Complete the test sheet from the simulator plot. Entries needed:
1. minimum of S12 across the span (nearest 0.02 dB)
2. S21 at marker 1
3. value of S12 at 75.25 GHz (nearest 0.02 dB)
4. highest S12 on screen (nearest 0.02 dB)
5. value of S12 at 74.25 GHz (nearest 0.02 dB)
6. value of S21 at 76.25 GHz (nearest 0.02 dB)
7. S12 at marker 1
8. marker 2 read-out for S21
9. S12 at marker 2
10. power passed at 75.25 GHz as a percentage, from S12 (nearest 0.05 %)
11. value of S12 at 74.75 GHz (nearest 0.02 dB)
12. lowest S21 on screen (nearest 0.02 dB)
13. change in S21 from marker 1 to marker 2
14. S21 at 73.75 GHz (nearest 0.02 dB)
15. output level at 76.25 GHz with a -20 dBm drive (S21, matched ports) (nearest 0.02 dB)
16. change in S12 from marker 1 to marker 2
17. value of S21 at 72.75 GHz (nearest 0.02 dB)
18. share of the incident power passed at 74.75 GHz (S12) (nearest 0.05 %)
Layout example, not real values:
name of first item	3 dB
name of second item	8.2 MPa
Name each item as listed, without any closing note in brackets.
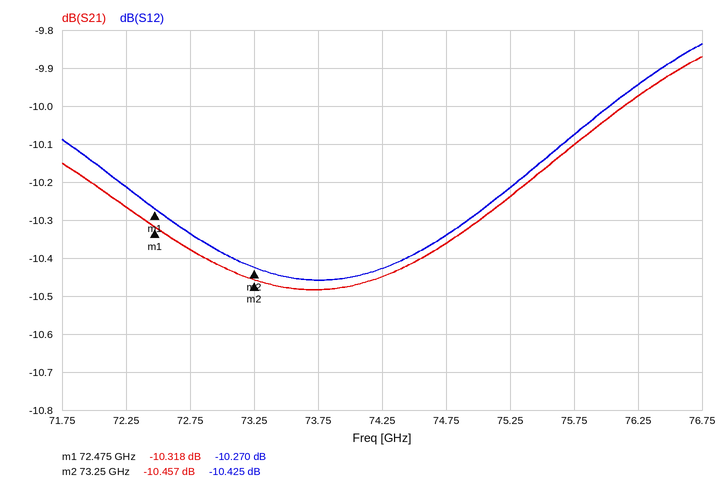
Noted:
minimum of S12 across the span	-10.46 dB
S21 at marker 1	-10.318 dB
value of S12 at 75.25 GHz	-10.22 dB
highest S12 on screen	-9.84 dB
value of S12 at 74.25 GHz	-10.42 dB
value of S21 at 76.25 GHz	-9.98 dB
S12 at marker 1	-10.270 dB
marker 2 read-out for S21	-10.457 dB
S12 at marker 2	-10.425 dB
power passed at 75.25 GHz as a percentage, from S12	9.50 %
value of S12 at 74.75 GHz	-10.34 dB
lowest S21 on screen	-10.48 dB
change in S21 from marker 1 to marker 2	-0.139 dB
S21 at 73.75 GHz	-10.48 dB
output level at 76.25 GHz with a -20 dBm drive (S21, matched ports)	-29.98 dBm
change in S12 from marker 1 to marker 2	-0.155 dB
value of S21 at 72.75 GHz	-10.38 dB
share of the incident power passed at 74.75 GHz (S12)	9.25 %
